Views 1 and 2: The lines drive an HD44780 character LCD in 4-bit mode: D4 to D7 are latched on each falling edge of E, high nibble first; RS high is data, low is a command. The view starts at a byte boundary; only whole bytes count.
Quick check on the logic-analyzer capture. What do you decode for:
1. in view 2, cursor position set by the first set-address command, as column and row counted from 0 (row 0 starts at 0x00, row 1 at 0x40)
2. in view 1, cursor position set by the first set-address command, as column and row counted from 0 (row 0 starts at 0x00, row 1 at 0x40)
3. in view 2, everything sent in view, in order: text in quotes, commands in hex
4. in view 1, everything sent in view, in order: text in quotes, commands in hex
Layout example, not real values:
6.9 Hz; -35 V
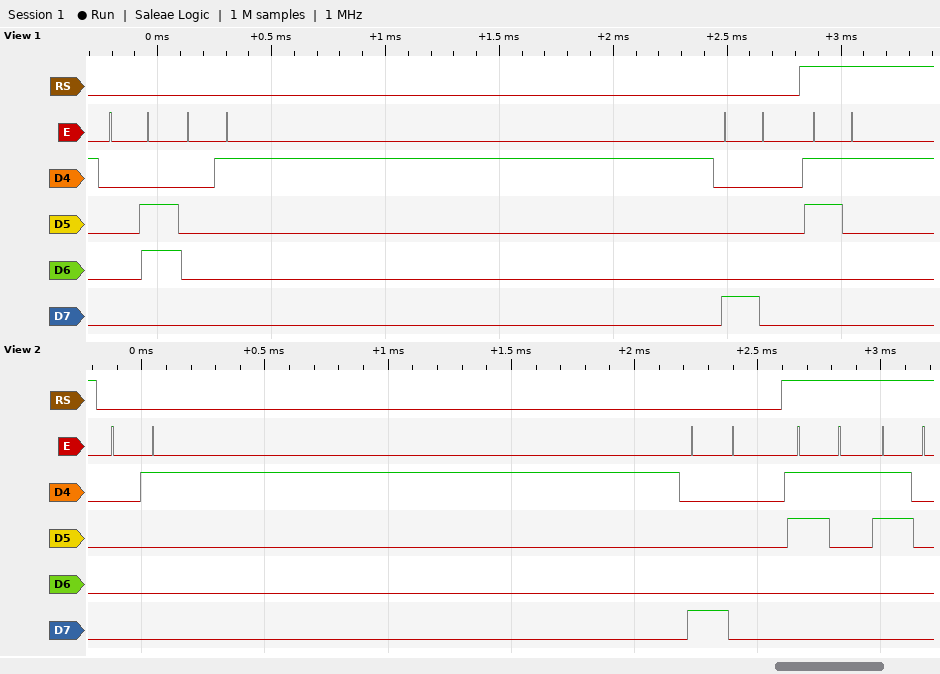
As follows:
column 0, row 0; column 0, row 0; 0x01 0x80 "10"; 0x06 0x01 0x80 "1"
